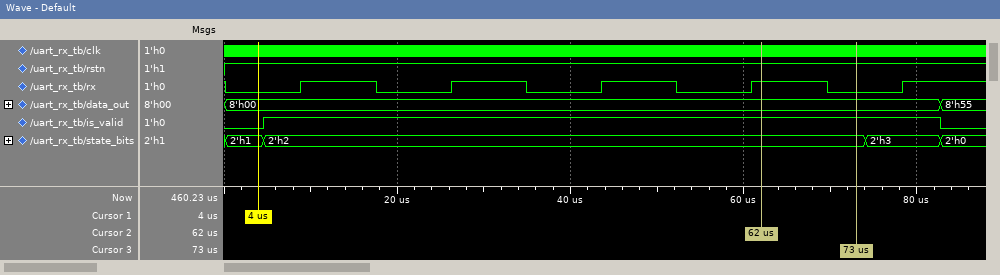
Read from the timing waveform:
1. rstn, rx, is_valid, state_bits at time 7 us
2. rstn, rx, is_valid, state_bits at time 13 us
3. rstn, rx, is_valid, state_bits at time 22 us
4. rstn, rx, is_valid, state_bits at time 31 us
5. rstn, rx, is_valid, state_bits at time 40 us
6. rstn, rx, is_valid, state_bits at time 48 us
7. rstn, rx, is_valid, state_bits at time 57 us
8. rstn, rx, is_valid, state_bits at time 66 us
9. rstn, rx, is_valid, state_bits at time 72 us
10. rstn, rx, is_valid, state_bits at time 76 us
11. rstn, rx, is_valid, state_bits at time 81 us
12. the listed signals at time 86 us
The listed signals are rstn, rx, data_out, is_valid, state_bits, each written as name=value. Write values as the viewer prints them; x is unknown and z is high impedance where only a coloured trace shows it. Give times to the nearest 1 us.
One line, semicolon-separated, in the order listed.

rstn=1, rx=0, is_valid=1, state_bits=2'h2; rstn=1, rx=1, is_valid=1, state_bits=2'h2; rstn=1, rx=0, is_valid=1, state_bits=2'h2; rstn=1, rx=1, is_valid=1, state_bits=2'h2; rstn=1, rx=0, is_valid=1, state_bits=2'h2; rstn=1, rx=1, is_valid=1, state_bits=2'h2; rstn=1, rx=0, is_valid=1, state_bits=2'h2; rstn=1, rx=1, is_valid=1, state_bits=2'h2; rstn=1, rx=0, is_valid=1, state_bits=2'h2; rstn=1, rx=0, is_valid=1, state_bits=2'h3; rstn=1, rx=1, is_valid=1, state_bits=2'h3; rstn=1, rx=1, data_out=8'h55, is_valid=0, state_bits=2'h0
